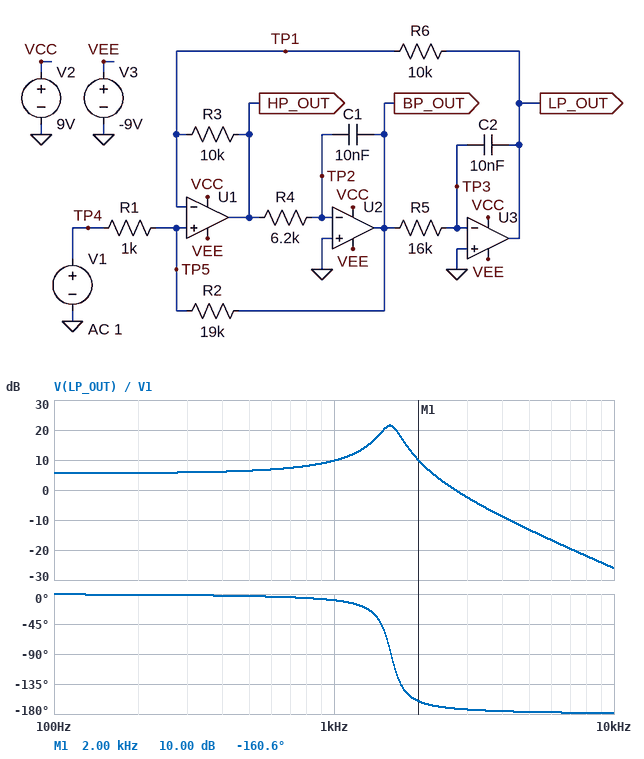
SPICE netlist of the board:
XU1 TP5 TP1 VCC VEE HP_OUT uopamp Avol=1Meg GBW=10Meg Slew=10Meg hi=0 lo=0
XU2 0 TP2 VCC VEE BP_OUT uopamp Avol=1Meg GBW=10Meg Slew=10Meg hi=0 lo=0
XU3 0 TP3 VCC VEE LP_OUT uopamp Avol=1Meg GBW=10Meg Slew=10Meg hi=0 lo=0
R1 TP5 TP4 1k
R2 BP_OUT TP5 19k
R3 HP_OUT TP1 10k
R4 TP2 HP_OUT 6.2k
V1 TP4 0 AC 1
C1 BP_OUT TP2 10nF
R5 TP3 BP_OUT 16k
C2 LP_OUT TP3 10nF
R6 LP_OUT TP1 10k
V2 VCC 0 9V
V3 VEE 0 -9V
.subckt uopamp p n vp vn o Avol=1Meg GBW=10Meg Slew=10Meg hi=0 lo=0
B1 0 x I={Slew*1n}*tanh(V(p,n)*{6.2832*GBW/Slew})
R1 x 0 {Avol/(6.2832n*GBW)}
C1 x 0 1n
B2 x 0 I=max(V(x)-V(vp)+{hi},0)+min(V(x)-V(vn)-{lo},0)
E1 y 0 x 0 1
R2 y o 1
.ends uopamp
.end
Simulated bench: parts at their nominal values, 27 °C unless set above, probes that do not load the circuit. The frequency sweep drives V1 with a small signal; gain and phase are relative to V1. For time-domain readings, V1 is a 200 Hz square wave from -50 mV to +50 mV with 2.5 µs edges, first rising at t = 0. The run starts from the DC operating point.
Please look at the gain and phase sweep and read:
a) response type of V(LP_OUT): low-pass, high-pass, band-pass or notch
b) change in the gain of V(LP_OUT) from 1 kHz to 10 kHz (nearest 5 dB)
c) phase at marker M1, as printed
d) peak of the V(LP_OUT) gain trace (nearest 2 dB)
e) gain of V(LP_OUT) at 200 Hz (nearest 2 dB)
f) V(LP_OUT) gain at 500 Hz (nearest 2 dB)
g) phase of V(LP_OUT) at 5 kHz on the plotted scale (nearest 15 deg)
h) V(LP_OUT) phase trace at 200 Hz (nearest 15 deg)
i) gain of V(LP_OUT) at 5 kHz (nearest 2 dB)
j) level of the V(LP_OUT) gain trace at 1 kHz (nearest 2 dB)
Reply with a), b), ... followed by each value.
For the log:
a) low-pass
b) -35 dB
c) -160.6 deg
d) 22 dB
e) 6 dB
f) 6 dB
g) -180 deg
h) 0 deg
i) -14 dB
j) 10 dB
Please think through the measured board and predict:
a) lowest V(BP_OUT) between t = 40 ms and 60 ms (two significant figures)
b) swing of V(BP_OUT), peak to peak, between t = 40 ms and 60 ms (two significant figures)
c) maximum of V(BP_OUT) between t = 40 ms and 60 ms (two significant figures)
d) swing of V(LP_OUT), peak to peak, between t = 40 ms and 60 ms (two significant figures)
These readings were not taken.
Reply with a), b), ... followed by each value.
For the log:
a) -240 mV
b) 480 mV
c) 240 mV
d) 450 mV
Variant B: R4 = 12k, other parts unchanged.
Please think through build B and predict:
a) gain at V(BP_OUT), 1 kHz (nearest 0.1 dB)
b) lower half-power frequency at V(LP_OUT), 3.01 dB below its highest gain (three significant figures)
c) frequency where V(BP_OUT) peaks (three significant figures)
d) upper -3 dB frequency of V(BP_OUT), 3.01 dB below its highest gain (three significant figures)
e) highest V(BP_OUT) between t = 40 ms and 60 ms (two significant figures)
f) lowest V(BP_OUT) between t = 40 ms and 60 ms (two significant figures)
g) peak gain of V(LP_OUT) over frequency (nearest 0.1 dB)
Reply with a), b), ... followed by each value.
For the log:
a) 17.3 dB
b) 1.08 kHz
c) 1.15 kHz
d) 1.22 kHz
e) 160 mV
f) -160 mV
g) 24.4 dB
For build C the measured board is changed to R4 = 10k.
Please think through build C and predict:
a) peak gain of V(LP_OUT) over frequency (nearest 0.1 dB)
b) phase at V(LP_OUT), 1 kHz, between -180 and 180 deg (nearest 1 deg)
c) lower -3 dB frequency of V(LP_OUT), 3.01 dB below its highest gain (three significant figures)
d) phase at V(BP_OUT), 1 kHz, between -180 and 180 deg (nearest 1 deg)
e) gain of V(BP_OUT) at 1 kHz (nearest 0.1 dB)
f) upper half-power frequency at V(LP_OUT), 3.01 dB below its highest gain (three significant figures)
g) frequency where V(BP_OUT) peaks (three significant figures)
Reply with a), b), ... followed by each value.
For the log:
a) 23.6 dB
b) -15 deg
c) 1.17 kHz
d) -105 deg
e) 14.0 dB
f) 1.33 kHz
g) 1.26 kHz
